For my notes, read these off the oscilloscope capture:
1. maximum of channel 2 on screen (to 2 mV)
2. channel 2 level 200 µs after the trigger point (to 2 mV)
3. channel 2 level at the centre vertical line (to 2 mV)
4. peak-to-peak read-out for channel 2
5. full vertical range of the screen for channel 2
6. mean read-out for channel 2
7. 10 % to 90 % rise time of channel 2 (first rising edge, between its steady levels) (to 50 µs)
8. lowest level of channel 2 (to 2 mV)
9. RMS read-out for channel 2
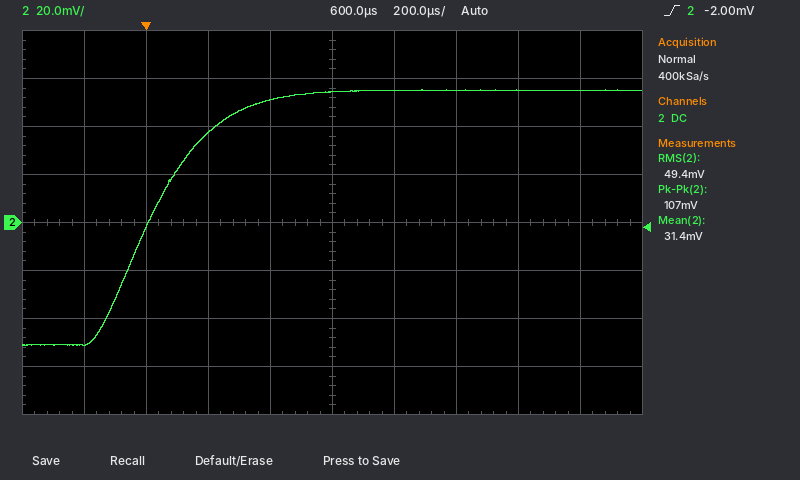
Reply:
56 mV
38 mV
54 mV
107 mV
160 mV
31.4 mV
400 µs
-52 mV
49.4 mV
